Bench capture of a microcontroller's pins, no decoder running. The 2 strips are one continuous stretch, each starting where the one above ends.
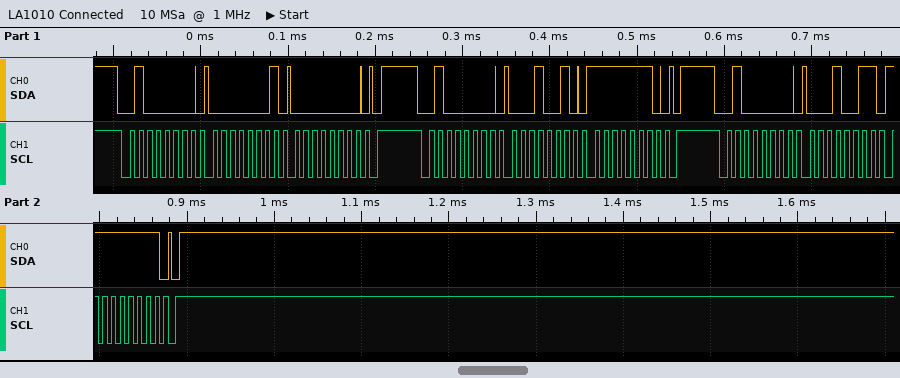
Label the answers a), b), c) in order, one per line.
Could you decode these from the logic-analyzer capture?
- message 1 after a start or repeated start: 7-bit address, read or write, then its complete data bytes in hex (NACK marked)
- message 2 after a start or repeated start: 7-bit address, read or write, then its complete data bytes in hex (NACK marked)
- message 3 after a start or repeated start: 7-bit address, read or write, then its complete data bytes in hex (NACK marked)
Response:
a) 0x20 write: 01 00
b) 0x20 write: 12 FE
c) 0x20 write: 13 FF
